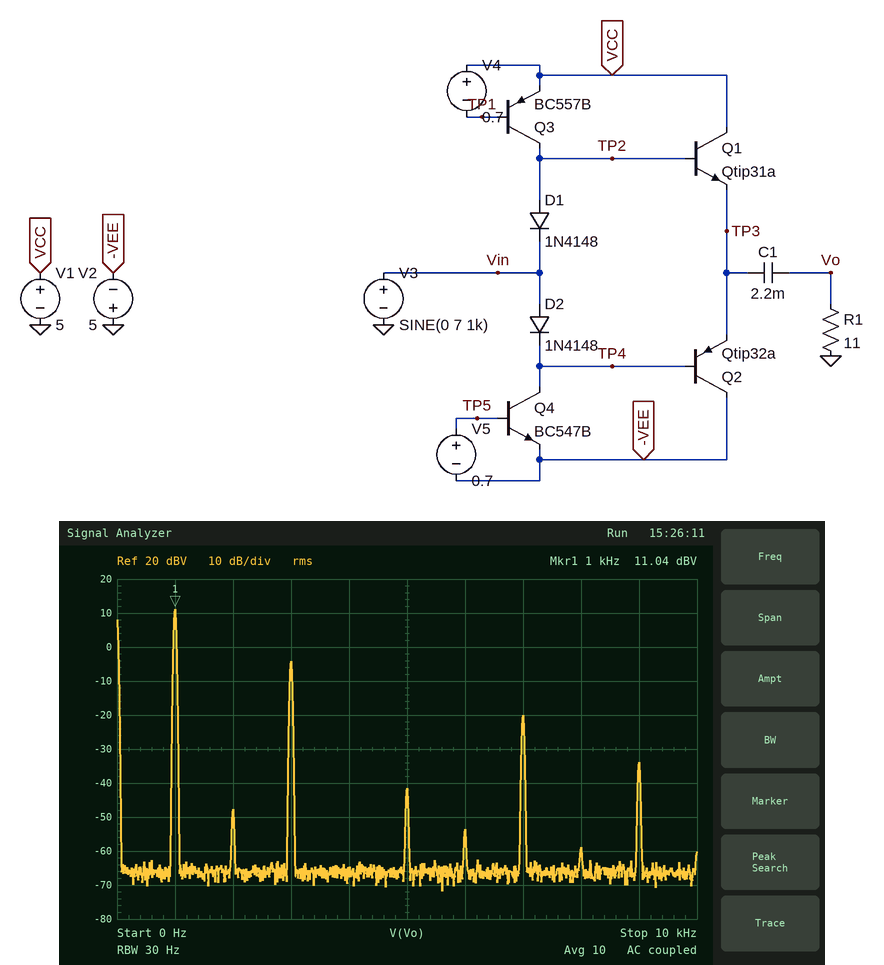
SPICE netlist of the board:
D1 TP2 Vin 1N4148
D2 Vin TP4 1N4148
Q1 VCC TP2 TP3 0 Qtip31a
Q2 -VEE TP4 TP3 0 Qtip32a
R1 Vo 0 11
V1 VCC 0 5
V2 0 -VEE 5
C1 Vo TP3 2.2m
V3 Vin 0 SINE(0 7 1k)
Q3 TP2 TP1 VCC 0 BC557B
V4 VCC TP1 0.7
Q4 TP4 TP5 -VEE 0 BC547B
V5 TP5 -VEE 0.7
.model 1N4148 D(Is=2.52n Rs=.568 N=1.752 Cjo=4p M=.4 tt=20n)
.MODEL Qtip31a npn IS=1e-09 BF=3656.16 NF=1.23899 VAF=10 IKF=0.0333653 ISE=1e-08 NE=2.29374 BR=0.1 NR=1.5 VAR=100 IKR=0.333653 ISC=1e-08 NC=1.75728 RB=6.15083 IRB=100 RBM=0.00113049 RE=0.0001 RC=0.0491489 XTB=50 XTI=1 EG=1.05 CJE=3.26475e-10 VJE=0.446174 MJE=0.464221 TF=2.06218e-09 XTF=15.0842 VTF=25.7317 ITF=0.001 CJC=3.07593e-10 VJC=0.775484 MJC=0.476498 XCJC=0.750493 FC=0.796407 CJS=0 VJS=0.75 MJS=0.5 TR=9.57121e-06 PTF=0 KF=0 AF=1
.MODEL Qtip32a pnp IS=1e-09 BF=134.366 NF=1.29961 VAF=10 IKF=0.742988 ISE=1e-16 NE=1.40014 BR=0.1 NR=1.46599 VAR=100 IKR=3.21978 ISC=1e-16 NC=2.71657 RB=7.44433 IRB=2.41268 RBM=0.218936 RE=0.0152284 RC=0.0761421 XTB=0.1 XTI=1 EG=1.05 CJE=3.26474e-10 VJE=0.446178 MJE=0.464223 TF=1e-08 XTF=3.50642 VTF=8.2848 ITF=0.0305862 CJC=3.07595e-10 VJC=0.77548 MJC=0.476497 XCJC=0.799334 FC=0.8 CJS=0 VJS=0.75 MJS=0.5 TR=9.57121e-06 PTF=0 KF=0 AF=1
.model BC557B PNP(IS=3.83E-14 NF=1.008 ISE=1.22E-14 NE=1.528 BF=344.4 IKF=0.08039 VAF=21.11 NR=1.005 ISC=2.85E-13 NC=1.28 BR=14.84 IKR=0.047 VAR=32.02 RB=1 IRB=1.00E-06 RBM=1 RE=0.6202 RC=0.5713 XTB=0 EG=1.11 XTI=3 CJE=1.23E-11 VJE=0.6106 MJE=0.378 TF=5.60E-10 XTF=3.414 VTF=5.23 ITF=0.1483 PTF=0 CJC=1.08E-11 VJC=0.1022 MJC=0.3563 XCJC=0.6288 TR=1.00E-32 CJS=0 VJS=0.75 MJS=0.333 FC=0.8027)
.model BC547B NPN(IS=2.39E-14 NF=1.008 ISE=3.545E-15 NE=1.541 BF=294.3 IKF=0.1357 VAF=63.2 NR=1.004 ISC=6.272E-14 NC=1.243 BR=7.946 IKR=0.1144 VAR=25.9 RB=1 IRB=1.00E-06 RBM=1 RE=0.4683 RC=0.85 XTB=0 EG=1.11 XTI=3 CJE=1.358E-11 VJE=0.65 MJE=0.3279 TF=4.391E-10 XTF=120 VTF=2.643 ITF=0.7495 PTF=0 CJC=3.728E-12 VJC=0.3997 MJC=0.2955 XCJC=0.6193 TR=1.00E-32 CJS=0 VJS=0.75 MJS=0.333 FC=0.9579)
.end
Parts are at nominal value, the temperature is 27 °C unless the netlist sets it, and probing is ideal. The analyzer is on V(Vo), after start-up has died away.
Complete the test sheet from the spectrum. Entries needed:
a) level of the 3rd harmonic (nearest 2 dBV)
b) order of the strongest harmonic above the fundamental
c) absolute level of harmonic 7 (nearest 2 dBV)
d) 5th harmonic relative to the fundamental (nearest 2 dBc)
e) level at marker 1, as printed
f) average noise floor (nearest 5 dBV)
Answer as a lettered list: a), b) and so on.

a) -4 dBV
b) 3
c) -20 dBV
d) -52 dBc
e) 11.04 dBV
f) -65 dBV
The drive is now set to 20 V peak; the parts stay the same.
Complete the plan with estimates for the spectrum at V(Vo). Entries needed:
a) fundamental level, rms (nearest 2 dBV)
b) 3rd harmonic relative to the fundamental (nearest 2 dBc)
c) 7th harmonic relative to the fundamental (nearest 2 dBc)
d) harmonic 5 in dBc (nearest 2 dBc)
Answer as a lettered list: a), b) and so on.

a) 12 dBV
b) -10 dBc
c) -20 dBc
d) -16 dBc
